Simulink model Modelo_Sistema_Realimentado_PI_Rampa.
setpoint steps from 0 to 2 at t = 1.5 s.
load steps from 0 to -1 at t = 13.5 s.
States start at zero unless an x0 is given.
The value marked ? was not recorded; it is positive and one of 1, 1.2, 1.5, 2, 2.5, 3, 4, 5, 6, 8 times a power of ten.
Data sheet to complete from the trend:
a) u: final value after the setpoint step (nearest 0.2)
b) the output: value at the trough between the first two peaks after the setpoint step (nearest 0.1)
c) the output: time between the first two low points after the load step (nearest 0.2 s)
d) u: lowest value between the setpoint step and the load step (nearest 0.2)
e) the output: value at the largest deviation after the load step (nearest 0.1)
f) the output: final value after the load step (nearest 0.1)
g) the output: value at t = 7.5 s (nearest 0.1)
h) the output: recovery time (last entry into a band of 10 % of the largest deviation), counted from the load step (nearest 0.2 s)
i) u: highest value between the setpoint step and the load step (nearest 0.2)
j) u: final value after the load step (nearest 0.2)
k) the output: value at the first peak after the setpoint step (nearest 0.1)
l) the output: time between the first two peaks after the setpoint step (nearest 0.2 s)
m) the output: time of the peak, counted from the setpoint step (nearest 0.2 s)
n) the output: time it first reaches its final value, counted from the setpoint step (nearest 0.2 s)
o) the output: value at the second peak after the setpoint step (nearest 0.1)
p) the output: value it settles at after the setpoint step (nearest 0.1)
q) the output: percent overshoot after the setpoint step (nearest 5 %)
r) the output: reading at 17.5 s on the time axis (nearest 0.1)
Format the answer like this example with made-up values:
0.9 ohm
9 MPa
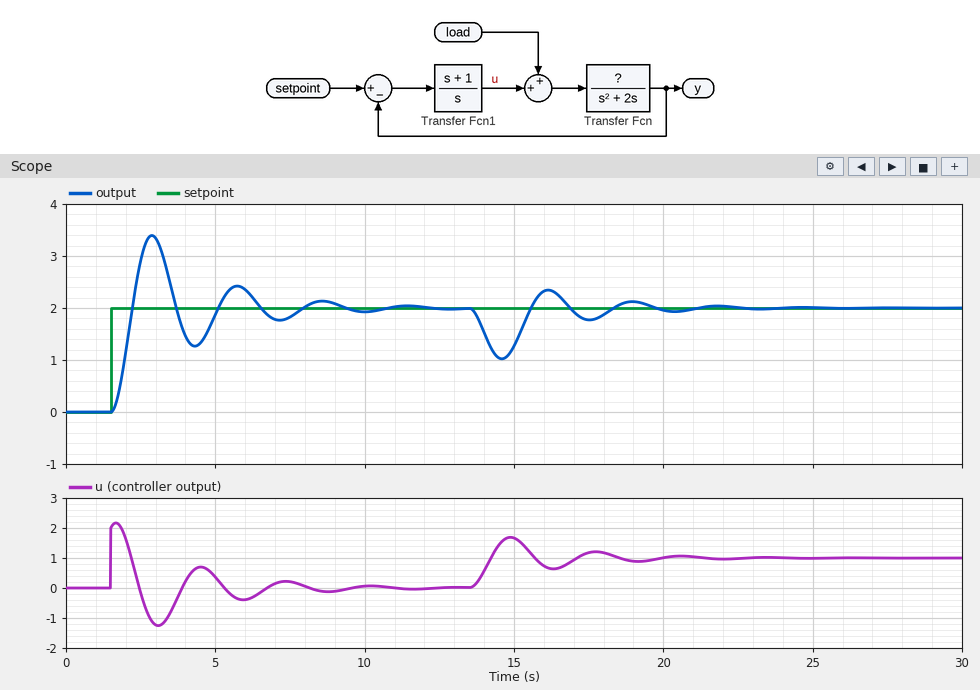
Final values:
0.0
1.3
3.0 s
-1.2
1.0
2.0
1.8
5.8 s
2.2
1.0
3.4
2.8 s
1.4 s
0.8 s
2.4
2.0
70 %
1.8
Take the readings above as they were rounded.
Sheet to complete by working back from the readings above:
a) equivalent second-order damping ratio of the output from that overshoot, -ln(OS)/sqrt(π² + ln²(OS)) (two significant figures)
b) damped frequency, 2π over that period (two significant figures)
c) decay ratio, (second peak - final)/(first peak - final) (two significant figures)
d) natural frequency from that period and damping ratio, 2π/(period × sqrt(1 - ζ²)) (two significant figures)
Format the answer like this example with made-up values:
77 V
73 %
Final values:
0.11
2.2 rad/s
0.29
2.3 rad/s
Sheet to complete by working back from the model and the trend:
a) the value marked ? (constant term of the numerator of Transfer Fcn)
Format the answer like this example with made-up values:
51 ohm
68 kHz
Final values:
6
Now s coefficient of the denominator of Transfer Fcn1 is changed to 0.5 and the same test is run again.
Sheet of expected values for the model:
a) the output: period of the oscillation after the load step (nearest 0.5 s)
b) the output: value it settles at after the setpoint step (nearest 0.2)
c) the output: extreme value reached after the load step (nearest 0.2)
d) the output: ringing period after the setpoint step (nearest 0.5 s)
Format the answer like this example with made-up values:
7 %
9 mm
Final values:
2.0 s
2.0
1.4
2.0 s
